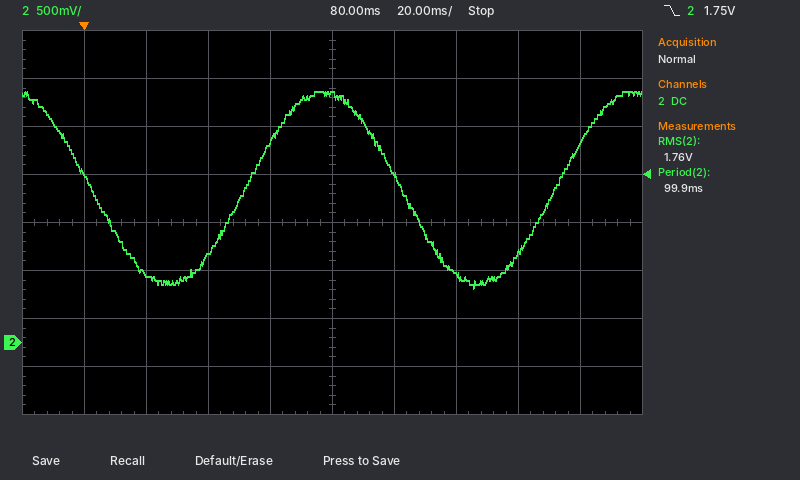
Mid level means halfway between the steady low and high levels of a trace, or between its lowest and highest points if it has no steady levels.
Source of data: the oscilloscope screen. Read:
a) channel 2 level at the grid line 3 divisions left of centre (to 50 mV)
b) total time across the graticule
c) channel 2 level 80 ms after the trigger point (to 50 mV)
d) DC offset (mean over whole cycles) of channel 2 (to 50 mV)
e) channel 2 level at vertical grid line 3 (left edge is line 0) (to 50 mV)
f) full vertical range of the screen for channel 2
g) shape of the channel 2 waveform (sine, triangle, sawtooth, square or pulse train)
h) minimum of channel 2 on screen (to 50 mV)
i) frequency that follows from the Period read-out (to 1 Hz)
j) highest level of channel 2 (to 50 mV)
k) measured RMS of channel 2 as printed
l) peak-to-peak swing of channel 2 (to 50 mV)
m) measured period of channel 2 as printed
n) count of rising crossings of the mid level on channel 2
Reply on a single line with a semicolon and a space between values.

700 mV; 200 ms; 2.60 V; 1.60 V; 900 mV; 4 V; sine; 550 mV; 10 Hz; 2.60 V; 1.76 V; 2.05 V; 99.9 ms; 2
